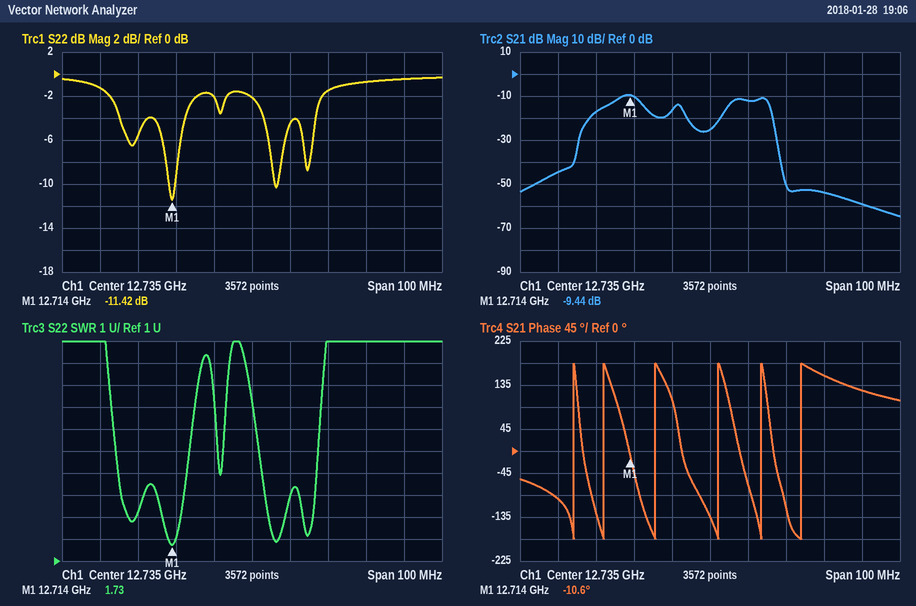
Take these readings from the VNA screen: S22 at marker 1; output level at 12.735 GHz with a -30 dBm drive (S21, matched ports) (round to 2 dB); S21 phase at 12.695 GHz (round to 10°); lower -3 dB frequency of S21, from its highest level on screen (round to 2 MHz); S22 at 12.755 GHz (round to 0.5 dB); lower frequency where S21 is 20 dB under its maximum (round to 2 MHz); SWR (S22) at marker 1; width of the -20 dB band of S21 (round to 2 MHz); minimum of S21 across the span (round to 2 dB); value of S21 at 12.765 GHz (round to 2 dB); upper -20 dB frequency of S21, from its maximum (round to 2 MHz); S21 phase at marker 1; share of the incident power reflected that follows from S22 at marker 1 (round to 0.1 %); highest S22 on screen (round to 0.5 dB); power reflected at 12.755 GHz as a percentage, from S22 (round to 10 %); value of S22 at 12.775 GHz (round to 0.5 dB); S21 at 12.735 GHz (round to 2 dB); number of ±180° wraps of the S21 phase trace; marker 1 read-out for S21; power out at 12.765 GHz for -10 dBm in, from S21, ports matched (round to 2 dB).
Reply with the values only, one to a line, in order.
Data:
-11.42 dB
-56 dBm
-100°
12.710 GHz
-1.5 dB
12.700 GHz
1.73
52 MHz
-64 dB
-54 dB
12.752 GHz
-10.6°
7.2 %
-0.5 dB
70 %
-0.5 dB
-26 dB
6
-9.44 dB
-64 dBm
